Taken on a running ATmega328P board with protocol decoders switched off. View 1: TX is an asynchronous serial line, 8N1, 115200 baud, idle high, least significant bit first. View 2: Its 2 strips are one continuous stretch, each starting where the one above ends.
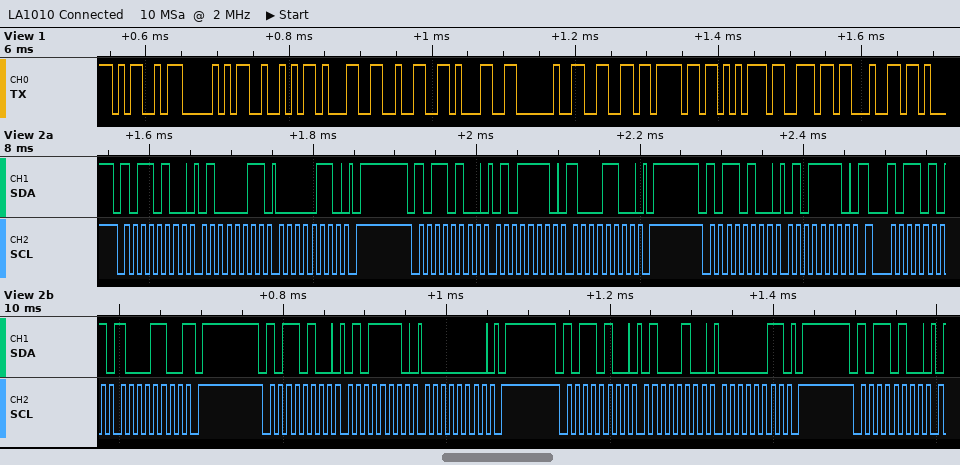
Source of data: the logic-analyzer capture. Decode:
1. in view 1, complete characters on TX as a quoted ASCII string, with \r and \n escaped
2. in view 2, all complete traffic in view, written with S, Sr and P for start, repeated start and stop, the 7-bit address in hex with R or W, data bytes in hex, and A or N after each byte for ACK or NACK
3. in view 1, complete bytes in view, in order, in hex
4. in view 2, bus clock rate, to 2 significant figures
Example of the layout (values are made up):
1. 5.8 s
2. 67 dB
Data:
1. "MPR121 found"
2. S 5AW A 43 A 06 A P S 5AW A 5E A 8C A P S 5AW A 5E A Sr 5AR A 8C N P S 5AW A 5E A 00 A P S 5AW A 44 A 03 A P S 5AW A
3. 0x4D 0x50 0x52 0x31 0x32 0x31 0x20 0x66 0x6F 0x75 0x6E 0x64
4. 100 kHz
